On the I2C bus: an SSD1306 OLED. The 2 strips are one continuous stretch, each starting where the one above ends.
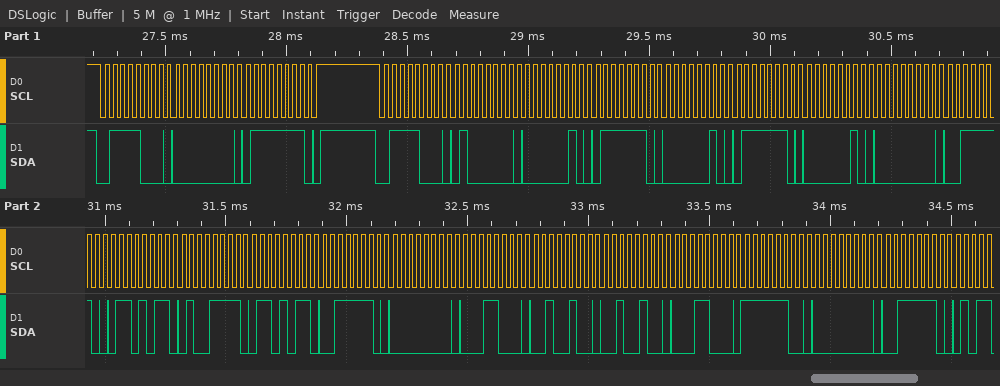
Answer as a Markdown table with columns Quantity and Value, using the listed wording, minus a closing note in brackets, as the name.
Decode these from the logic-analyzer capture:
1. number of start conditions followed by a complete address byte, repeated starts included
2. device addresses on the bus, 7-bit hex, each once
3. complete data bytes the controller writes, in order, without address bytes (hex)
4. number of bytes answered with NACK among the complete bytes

| Quantity | Value |
|---|---|
| number of start conditions followed by a complete address byte, repeated starts included | 2 |
| device addresses on the bus, 7-bit hex, each once | 0x3C |
| complete data bytes the controller writes, in order, without address bytes | 00 7F 40 02 7E 02 7E 02 00 3E 6B 4F 6B 3E 00 18 24 24 18 FC 00 3E |
| number of bytes answered with NACK among the complete bytes | 0 |
